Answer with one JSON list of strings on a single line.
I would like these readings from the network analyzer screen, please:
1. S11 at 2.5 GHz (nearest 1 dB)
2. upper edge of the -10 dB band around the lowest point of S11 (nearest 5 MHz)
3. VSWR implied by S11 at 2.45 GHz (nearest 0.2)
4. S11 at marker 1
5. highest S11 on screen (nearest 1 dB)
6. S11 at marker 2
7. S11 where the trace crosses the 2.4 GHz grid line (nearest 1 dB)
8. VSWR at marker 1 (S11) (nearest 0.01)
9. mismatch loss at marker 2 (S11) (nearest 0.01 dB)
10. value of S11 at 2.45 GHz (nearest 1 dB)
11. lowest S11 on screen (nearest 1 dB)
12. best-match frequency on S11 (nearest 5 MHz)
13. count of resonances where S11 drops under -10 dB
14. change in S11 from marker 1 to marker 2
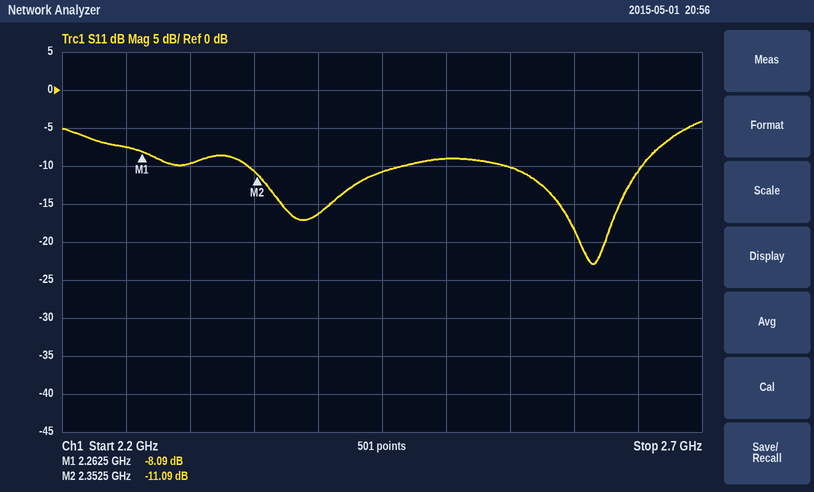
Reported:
["-9 dB", "2.655 GHz", "1.8", "-8.09 dB", "-4 dB", "-11.09 dB", "-16 dB", "2.30", "0.35 dB", "-11 dB", "-23 dB", "2.615 GHz", "2", "-3.00 dB"]
